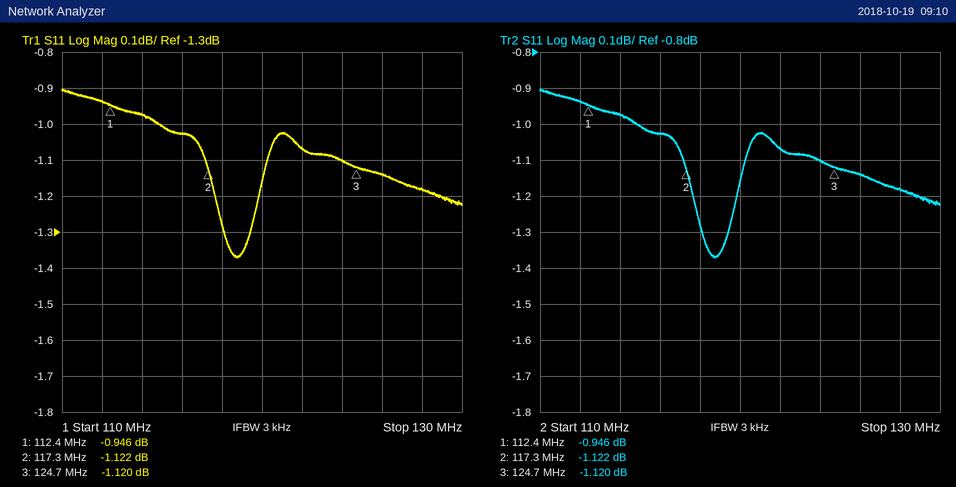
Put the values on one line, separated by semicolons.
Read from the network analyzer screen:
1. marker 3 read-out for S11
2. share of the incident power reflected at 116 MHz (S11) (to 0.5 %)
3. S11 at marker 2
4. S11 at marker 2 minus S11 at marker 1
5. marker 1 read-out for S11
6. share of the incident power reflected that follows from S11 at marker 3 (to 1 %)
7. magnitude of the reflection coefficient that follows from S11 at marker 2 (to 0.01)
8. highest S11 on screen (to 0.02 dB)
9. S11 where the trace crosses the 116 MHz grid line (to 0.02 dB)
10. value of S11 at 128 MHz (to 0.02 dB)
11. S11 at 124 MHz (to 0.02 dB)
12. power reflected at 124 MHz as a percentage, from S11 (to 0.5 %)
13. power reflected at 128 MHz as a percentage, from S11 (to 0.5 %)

-1.120 dB; 79.0 %; -1.122 dB; -0.176 dB; -0.946 dB; 77 %; 0.88; -0.90 dB; -1.02 dB; -1.18 dB; -1.10 dB; 77.5 %; 76.0 %
